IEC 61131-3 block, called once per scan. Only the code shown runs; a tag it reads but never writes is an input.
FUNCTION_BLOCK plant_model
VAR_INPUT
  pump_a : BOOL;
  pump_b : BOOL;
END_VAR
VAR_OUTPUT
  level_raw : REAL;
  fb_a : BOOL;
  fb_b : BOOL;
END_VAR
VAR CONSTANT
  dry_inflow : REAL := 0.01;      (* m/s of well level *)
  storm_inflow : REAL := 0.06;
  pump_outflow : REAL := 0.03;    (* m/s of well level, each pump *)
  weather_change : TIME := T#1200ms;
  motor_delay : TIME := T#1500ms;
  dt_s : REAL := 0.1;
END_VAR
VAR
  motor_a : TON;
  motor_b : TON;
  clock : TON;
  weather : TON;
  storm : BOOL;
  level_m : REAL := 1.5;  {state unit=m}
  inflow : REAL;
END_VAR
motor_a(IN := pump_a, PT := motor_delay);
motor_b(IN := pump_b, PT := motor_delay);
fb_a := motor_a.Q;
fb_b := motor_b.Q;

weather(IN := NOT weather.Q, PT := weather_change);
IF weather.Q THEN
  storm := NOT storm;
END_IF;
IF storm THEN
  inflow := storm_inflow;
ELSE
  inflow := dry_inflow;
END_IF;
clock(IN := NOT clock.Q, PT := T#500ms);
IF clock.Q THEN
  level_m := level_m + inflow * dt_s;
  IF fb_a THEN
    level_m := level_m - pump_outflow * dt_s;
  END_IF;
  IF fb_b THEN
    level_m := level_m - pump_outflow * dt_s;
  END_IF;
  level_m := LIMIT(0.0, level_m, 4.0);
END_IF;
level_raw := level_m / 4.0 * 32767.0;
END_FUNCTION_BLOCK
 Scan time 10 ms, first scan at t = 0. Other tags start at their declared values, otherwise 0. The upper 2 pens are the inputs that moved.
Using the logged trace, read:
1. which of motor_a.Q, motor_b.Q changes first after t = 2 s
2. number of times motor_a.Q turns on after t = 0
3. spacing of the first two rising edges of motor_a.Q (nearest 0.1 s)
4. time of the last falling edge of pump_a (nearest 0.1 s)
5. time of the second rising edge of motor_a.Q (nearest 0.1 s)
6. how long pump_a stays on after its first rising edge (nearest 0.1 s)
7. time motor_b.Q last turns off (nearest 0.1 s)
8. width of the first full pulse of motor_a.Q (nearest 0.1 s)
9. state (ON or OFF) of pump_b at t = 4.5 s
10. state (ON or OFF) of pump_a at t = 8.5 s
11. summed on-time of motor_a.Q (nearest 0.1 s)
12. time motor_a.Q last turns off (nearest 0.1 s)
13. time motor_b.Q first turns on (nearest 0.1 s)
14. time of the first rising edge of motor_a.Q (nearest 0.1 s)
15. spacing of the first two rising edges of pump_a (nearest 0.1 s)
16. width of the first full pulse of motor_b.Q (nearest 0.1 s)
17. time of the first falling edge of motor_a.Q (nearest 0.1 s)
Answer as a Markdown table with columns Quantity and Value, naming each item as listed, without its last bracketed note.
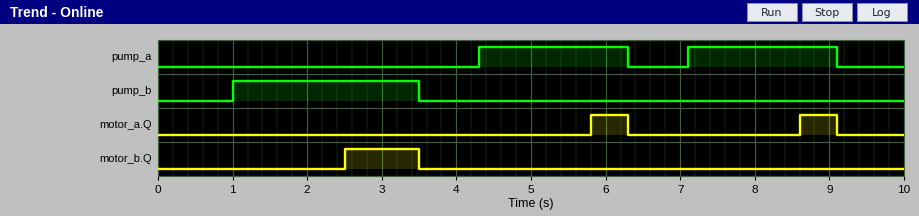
| Quantity | Value |
|---|---|
| which of motor_a.Q, motor_b.Q changes first after t = 2 s | motor_b.Q |
| number of times motor_a.Q turns on after t = 0 | 2 |
| spacing of the first two rising edges of motor_a.Q | 2.8 s |
| time of the last falling edge of pump_a | 9.1 s |
| time of the second rising edge of motor_a.Q | 8.6 s |
| how long pump_a stays on after its first rising edge | 2.0 s |
| time motor_b.Q last turns off | 3.5 s |
| width of the first full pulse of motor_a.Q | 0.5 s |
| state (ON or OFF) of pump_b at t = 4.5 s | OFF |
| state (ON or OFF) of pump_a at t = 8.5 s | ON |
| summed on-time of motor_a.Q | 1.0 s |
| time motor_a.Q last turns off | 9.1 s |
| time motor_b.Q first turns on | 2.5 s |
| time of the first rising edge of motor_a.Q | 5.8 s |
| spacing of the first two rising edges of pump_a | 2.8 s |
| width of the first full pulse of motor_b.Q | 1.0 s |
| time of the first falling edge of motor_a.Q | 6.3 s |
